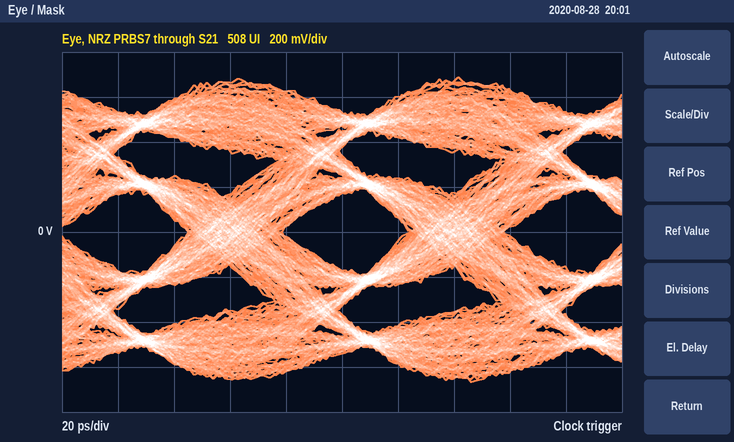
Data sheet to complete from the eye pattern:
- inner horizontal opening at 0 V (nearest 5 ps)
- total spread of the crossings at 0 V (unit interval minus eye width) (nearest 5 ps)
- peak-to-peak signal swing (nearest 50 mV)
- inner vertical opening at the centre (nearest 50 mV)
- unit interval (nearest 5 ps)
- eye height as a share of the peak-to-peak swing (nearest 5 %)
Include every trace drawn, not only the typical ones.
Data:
45 ps
35 ps
1.35 V
350 mV
80 ps
25 %
